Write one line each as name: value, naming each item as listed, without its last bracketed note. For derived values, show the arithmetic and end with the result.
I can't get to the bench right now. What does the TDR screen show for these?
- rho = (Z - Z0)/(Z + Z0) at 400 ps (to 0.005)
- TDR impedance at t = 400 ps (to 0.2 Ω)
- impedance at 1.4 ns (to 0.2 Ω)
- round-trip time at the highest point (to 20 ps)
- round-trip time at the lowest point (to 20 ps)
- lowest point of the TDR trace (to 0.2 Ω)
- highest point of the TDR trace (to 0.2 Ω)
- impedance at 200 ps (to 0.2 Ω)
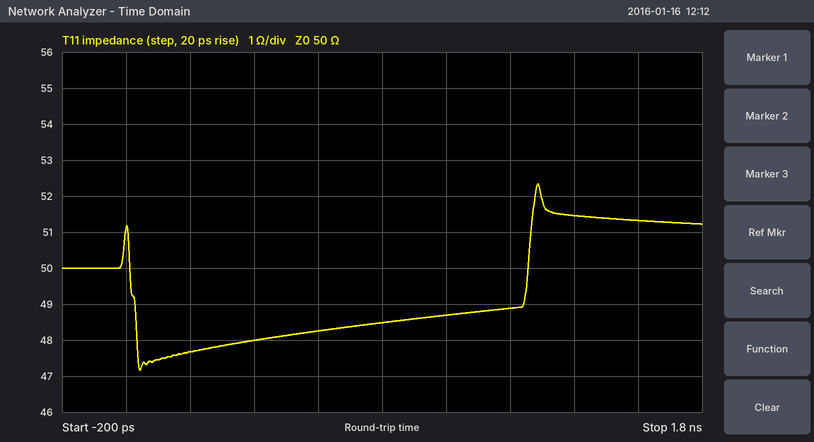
rho = (Z - Z0)/(Z + Z0) at 400 ps: (48 − 50)/(48 + 50) ≈ -0.020
TDR impedance at t = 400 ps: 48.0 Ω
impedance at 1.4 ns: 51.4 Ω
round-trip time at the highest point: 1.28 ns
round-trip time at the lowest point: 40 ps
lowest point of the TDR trace: 47.2 Ω
highest point of the TDR trace: 52.4 Ω
impedance at 200 ps: 47.6 Ω
